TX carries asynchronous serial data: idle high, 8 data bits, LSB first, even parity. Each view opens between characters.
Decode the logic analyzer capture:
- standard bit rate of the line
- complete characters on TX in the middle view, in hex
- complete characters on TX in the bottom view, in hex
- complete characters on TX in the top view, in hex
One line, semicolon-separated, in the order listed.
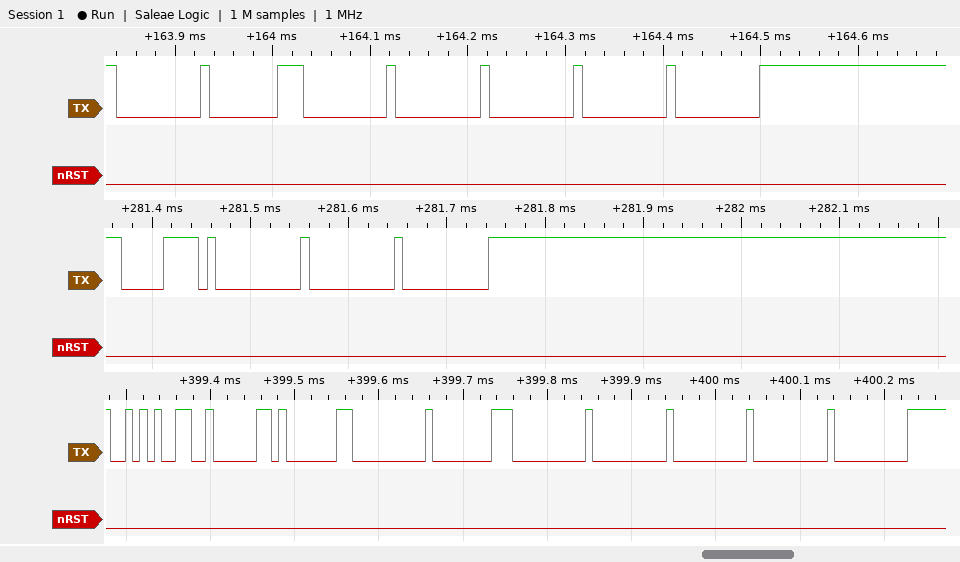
115200 baud; F0, 00, 00, 00; 2A, 02, 01, 00, 80, 00, 00, 00, 00, 00; 00, 80, 00, 00, 00, 00, 00
